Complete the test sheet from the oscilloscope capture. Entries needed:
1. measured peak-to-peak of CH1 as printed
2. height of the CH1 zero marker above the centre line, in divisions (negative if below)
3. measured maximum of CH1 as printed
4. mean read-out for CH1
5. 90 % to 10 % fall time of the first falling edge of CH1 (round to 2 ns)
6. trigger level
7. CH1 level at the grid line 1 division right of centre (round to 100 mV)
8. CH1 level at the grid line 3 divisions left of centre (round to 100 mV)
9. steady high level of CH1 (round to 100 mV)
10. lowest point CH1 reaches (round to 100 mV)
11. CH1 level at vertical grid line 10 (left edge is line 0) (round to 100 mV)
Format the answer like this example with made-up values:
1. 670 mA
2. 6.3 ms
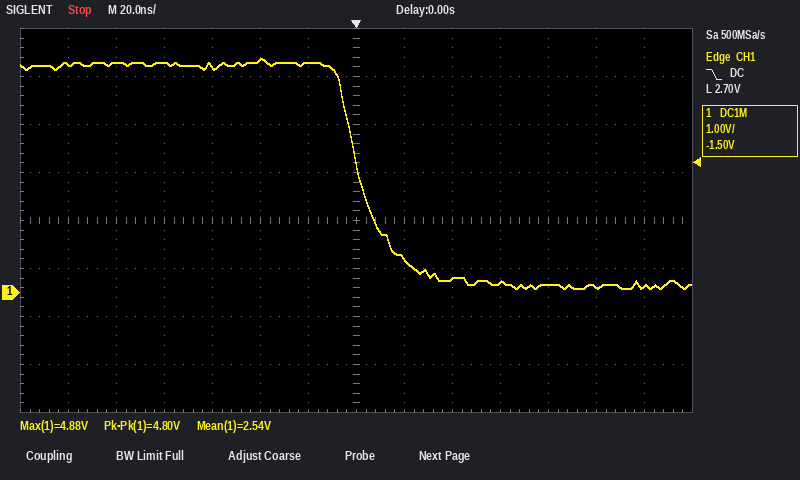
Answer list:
1. 4.80 V
2. -1.5 div
3. 4.88 V
4. 2.54 V
5. 28 ns
6. 2.70 V
7. 700 mV
8. 4.7 V
9. 4.8 V
10. 100 mV
11. 200 mV
